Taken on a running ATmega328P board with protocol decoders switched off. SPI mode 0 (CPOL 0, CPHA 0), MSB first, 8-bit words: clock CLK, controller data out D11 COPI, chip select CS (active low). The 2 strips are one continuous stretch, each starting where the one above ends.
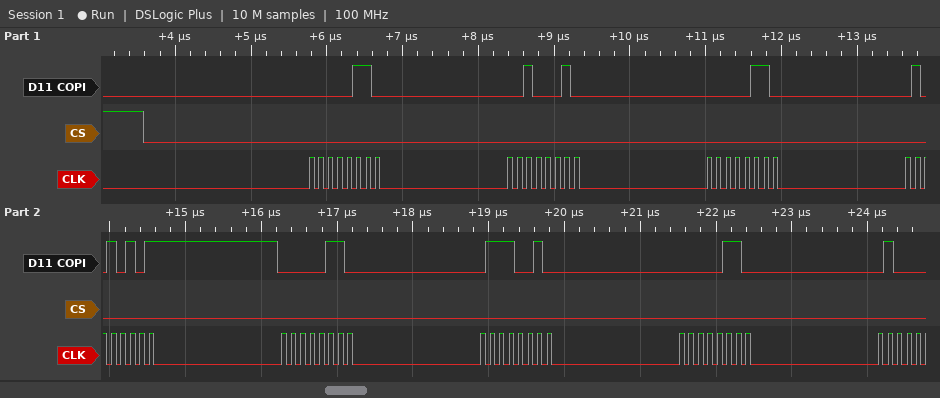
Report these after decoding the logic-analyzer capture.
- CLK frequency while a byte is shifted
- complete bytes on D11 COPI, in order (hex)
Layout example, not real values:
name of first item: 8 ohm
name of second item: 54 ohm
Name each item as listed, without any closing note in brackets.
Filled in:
CLK frequency while a byte is shifted: 8 MHz
complete bytes on D11 COPI, in order: 06 22 06 55 06 72 06
